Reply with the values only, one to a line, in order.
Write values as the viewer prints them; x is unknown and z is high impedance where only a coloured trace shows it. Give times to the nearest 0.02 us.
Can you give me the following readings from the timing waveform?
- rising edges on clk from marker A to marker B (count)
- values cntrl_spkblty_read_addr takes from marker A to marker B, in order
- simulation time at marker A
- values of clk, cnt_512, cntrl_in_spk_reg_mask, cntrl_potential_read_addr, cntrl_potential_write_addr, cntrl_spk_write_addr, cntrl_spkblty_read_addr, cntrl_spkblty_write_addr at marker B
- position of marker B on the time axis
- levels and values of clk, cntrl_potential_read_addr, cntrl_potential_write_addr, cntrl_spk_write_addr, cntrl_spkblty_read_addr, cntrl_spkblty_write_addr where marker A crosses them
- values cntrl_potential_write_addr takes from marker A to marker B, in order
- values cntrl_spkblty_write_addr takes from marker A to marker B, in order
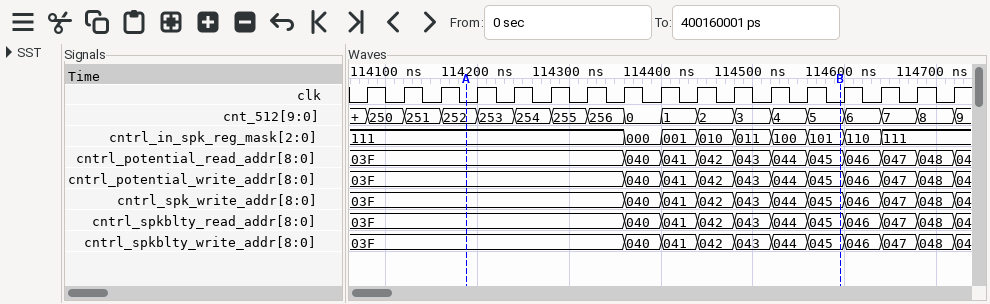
10
03F, 040, 041, 042, 043, 044, 045
114.18 us
clk=0, cnt_512=5, cntrl_in_spk_reg_mask=101, cntrl_potential_read_addr=045, cntrl_potential_write_addr=045, cntrl_spk_write_addr=045, cntrl_spkblty_read_addr=045, cntrl_spkblty_write_addr=045
114.6 us
clk=0, cntrl_potential_read_addr=03F, cntrl_potential_write_addr=03F, cntrl_spk_write_addr=03F, cntrl_spkblty_read_addr=03F, cntrl_spkblty_write_addr=03F
03F, 040, 041, 042, 043, 044, 045
03F, 040, 041, 042, 043, 044, 045
